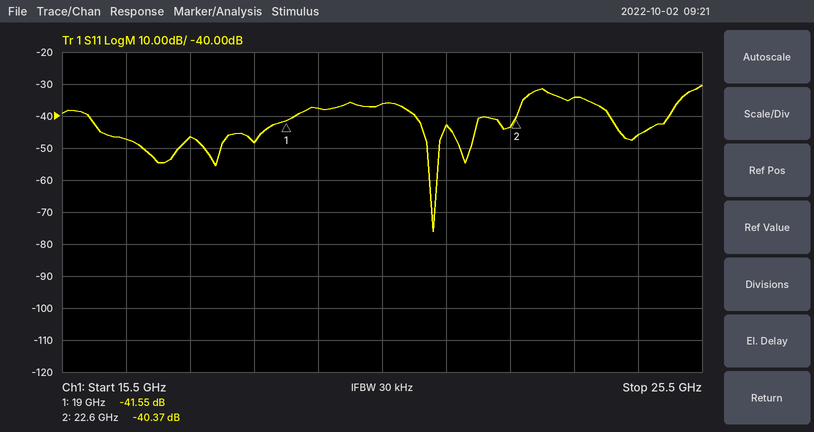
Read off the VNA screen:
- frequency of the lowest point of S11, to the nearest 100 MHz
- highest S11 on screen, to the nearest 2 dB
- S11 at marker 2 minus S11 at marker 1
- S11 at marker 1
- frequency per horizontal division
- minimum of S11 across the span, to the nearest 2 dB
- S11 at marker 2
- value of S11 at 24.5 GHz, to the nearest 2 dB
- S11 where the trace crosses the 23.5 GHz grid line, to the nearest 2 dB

21.3 GHz
-30 dB
1.18 dB
-41.55 dB
1 GHz
-76 dB
-40.37 dB
-46 dB
-34 dB
